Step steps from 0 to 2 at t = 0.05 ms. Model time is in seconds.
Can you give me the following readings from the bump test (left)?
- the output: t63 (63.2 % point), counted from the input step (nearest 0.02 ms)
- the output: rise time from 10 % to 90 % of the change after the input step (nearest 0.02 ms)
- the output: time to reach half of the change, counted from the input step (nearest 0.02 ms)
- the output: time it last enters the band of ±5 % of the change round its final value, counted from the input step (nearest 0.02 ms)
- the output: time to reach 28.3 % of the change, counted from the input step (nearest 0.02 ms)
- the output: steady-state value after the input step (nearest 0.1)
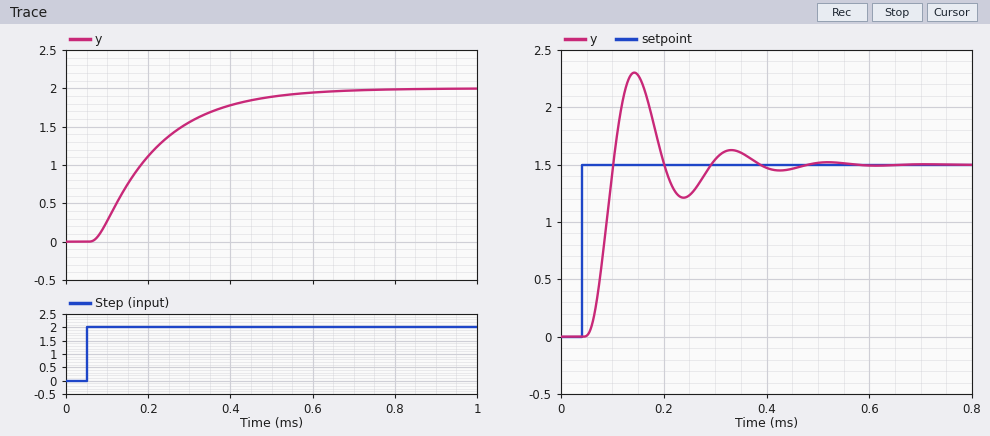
0.18 ms
0.32 ms
0.14 ms
0.46 ms
0.08 ms
2.0
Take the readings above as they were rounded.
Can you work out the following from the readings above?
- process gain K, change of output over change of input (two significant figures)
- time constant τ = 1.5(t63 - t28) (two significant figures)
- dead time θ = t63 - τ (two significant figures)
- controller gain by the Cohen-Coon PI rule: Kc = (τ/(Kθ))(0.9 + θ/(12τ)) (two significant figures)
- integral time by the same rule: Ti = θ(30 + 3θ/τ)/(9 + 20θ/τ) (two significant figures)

1.0
0.15 ms
0.030 ms
4.6
0.071 ms
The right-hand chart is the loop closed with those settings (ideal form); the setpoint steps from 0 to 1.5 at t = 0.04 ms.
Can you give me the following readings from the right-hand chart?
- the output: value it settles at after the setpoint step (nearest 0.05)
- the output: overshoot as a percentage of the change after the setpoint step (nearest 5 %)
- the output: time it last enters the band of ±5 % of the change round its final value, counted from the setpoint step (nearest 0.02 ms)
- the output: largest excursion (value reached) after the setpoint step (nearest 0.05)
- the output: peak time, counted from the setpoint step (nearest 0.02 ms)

1.50
55 %
0.32 ms
2.30
0.10 ms
